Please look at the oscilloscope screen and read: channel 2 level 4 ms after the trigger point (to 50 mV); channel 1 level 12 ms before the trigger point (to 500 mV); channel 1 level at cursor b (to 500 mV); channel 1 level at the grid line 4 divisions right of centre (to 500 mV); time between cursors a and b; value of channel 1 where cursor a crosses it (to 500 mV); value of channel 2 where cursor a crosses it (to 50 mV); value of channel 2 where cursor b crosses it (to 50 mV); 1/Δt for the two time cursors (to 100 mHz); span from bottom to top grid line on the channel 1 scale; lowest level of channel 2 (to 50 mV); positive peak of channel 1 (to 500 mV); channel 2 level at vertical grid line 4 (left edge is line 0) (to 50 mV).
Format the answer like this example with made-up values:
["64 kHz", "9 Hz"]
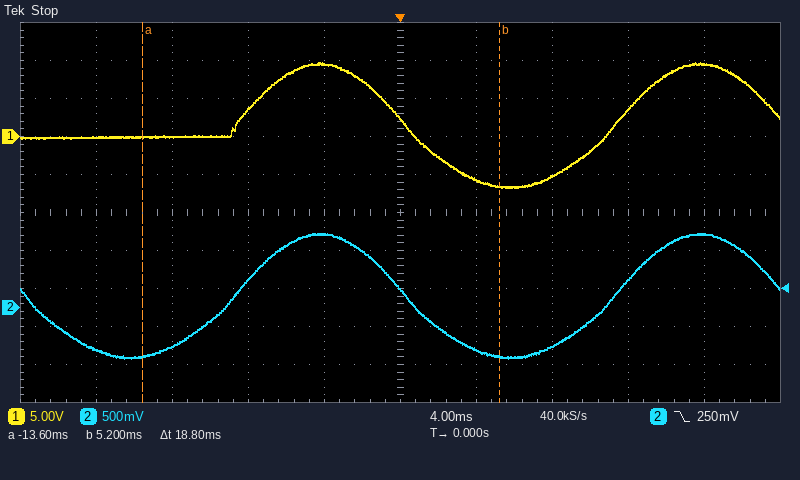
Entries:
["-550 mV", "0.0 V", "-6.5 V", "9.5 V", "18.8 ms", "0.0 V", "-650 mV", "-650 mV", "53.2 Hz", "50 V", "-650 mV", "9.5 V", "950 mV"]
